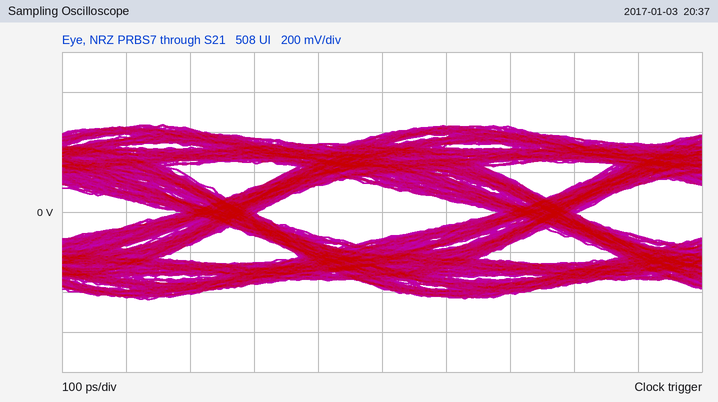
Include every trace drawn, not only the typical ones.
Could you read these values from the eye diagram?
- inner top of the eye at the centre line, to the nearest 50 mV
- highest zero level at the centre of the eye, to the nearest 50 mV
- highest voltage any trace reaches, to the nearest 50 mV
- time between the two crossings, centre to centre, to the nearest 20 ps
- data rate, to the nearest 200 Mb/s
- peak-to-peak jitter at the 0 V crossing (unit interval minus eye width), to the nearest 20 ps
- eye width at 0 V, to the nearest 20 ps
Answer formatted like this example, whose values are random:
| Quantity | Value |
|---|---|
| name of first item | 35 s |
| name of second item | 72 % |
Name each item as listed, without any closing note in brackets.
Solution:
| Quantity | Value |
|---|---|
| inner top of the eye at the centre line, to the nearest 50 mV | 150 mV |
| highest zero level at the centre of the eye, to the nearest 50 mV | -150 mV |
| highest voltage any trace reaches, to the nearest 50 mV | 450 mV |
| time between the two crossings, centre to centre, to the nearest 20 ps | 500 ps |
| data rate, to the nearest 200 Mb/s | 2.0 Gb/s |
| peak-to-peak jitter at the 0 V crossing (unit interval minus eye width), to the nearest 20 ps | 120 ps |
| eye width at 0 V, to the nearest 20 ps | 380 ps |
